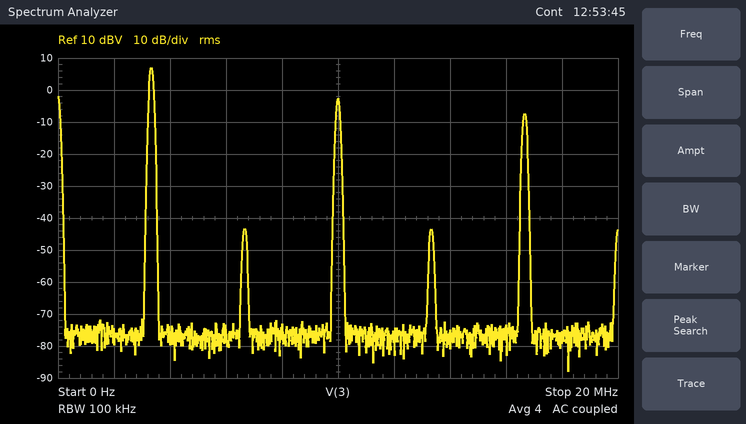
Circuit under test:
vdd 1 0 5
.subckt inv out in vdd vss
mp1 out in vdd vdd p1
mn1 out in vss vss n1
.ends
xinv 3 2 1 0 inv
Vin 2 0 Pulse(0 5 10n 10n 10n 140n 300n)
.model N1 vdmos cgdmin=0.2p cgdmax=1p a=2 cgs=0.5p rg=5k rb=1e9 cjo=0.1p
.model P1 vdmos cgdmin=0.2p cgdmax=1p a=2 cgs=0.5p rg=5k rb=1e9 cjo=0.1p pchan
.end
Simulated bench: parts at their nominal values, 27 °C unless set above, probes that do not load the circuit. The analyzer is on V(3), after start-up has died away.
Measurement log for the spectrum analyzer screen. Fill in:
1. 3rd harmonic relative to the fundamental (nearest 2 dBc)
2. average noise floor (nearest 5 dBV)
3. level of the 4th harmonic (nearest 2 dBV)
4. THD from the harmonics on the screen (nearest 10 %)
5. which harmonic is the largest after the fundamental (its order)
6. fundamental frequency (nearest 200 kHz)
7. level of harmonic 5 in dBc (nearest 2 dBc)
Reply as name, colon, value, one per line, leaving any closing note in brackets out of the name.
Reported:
3rd harmonic relative to the fundamental: -10 dBc
average noise floor: -75 dBV
level of the 4th harmonic: -44 dBV
THD from the harmonics on the screen: 40 %
which harmonic is the largest after the fundamental: 3
fundamental frequency: 3.4 MHz
level of harmonic 5 in dBc: -14 dBc
